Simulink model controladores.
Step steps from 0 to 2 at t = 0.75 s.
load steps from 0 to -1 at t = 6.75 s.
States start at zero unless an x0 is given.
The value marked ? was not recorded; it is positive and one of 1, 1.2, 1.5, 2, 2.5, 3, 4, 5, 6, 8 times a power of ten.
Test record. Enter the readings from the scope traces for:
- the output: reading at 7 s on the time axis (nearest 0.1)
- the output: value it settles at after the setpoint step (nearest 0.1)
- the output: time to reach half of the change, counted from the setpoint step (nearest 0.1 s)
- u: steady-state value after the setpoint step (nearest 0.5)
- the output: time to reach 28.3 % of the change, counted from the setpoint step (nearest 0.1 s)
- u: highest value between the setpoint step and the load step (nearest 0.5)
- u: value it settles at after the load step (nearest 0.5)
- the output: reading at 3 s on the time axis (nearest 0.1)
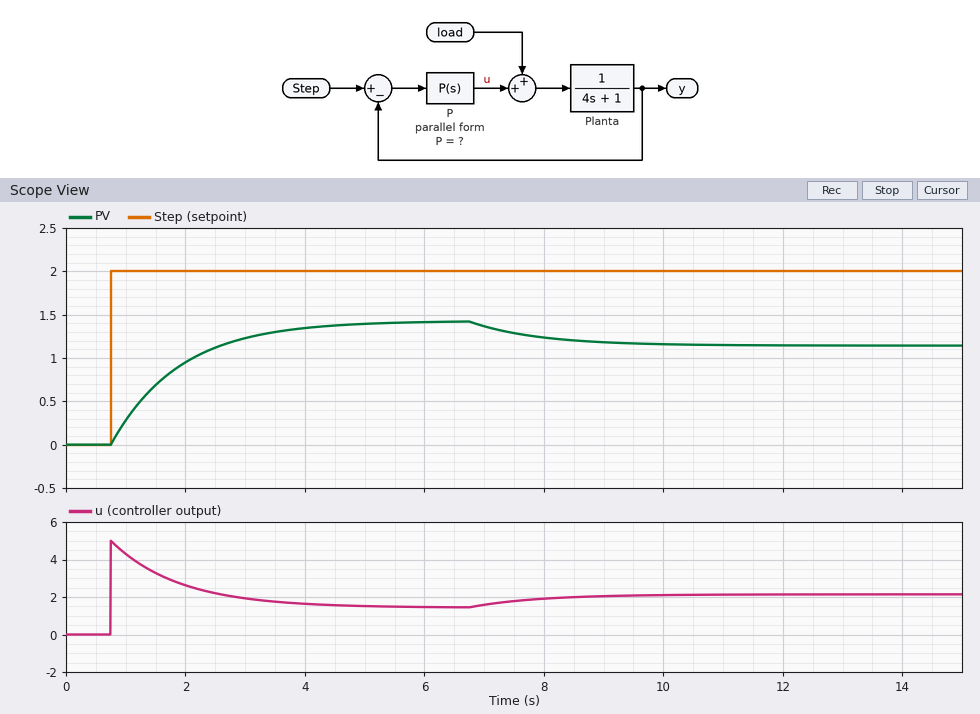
1.4
1.4
0.8 s
1.5
0.4 s
5.0
2.0
1.2
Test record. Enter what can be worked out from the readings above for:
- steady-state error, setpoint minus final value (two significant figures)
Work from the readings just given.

0.60
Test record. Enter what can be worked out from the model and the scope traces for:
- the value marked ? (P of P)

2.5
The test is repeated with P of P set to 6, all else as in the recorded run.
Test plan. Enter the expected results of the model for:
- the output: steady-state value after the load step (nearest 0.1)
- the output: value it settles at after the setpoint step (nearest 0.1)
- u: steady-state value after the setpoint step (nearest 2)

1.6
1.7
2
